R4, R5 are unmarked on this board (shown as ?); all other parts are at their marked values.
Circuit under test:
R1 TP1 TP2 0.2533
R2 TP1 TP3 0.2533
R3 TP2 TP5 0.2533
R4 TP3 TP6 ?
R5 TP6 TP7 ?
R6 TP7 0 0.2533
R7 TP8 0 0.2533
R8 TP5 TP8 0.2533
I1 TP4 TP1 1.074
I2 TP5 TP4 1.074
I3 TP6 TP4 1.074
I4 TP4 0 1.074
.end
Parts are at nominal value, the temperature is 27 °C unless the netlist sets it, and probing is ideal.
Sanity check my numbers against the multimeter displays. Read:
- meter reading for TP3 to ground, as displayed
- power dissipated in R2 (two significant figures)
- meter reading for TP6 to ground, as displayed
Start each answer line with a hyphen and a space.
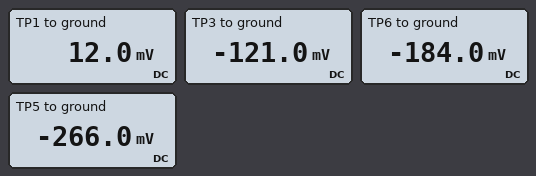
- -121.0 mV
- 70 mW
- -184.0 mV
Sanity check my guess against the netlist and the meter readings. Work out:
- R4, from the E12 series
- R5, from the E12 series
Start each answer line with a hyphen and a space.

- 0.12 Ω
- 0.082 Ω
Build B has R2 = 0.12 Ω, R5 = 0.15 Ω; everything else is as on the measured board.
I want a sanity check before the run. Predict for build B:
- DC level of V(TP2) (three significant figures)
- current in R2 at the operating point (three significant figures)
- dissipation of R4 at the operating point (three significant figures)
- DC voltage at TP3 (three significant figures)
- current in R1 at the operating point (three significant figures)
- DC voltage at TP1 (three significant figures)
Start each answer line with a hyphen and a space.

- -176 mV
- 590 mA
- 41.8 mW
- -124 mV
- 484 mA
- -53.6 mV
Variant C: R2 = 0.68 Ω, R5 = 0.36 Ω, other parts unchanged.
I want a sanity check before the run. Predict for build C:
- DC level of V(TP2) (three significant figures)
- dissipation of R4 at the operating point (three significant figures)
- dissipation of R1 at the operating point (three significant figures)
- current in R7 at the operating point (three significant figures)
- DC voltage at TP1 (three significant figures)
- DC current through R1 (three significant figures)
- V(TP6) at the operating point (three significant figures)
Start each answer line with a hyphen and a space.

- -105 mV
- 29.5 mW
- 84.7 mW
- 496 mA
- 41.9 mV
- 578 mA
- -355 mV
